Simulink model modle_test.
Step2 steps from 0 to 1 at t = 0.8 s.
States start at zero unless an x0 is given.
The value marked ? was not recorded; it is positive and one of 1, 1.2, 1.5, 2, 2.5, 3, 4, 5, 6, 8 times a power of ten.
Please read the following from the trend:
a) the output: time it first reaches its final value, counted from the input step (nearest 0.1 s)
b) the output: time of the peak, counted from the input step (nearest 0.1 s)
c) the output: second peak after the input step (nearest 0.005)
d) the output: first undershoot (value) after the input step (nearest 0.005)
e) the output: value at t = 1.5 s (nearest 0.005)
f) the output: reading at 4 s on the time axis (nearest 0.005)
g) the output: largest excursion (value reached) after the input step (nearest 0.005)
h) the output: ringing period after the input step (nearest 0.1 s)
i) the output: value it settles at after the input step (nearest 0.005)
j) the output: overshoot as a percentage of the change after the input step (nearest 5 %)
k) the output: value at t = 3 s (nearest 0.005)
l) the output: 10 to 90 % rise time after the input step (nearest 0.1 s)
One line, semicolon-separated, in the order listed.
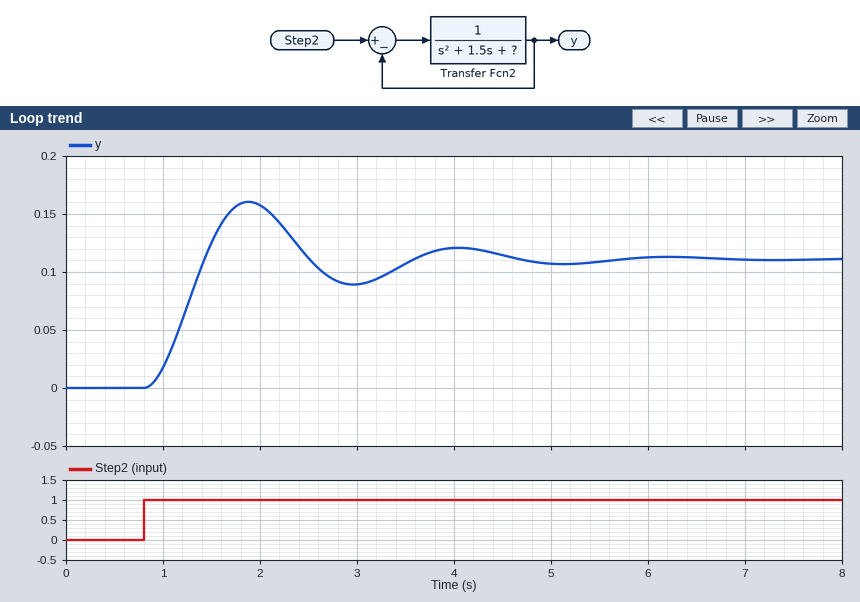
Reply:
0.6 s; 1.1 s; 0.120; 0.090; 0.125; 0.120; 0.160; 2.2 s; 0.110; 45 %; 0.090; 0.4 s
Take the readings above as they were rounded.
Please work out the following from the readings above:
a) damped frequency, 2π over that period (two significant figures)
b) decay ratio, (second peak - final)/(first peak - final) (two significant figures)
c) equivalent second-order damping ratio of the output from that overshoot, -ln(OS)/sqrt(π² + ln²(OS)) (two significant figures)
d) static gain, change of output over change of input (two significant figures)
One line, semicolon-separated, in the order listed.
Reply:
2.9 rad/s; 0.20; 0.25; 0.11
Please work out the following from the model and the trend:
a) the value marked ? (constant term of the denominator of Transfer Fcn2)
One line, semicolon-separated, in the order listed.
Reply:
8
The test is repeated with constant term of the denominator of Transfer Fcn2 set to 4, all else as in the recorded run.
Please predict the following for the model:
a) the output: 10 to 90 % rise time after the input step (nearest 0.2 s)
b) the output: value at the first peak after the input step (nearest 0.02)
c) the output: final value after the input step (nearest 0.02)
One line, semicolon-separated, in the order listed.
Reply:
0.6 s; 0.26; 0.20
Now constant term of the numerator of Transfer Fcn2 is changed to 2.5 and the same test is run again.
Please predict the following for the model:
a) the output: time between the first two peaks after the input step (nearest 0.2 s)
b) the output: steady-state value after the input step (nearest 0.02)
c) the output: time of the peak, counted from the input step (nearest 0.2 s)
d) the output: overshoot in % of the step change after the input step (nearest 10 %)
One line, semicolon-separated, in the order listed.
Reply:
2.0 s; 0.24; 1.0 s; 50 %
